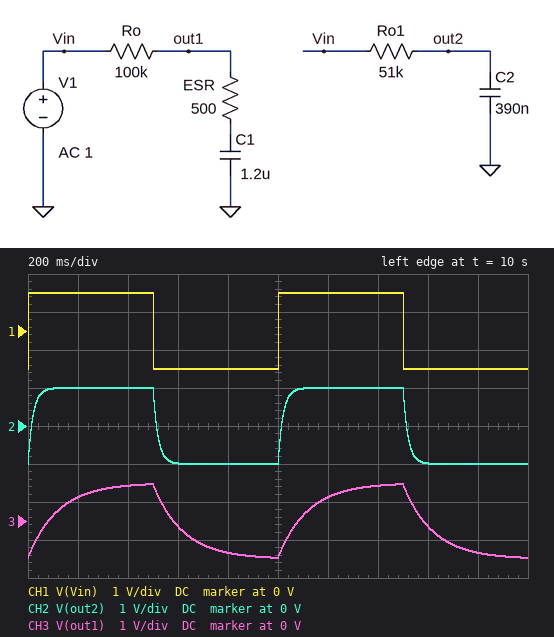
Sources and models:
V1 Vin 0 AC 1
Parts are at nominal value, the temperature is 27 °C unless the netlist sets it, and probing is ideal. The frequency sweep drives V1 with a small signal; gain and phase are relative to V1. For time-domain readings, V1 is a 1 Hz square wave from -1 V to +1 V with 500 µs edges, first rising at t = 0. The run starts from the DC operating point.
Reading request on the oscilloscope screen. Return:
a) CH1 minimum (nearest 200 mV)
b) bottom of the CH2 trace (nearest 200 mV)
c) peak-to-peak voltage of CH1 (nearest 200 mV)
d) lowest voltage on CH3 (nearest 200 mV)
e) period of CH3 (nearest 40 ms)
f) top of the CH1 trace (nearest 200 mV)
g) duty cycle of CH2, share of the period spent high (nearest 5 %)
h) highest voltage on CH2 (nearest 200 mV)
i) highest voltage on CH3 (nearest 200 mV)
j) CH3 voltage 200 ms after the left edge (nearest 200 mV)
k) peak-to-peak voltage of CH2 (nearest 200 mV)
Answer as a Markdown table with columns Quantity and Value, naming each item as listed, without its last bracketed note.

| Quantity | Value |
|---|---|
| CH1 minimum | -1.0 V |
| bottom of the CH2 trace | -1.0 V |
| peak-to-peak voltage of CH1 | 2.0 V |
| lowest voltage on CH3 | -1.0 V |
| period of CH3 | 1.00 s |
| top of the CH1 trace | 1.0 V |
| duty cycle of CH2, share of the period spent high | 50 % |
| highest voltage on CH2 | 1.0 V |
| highest voltage on CH3 | 1.0 V |
| CH3 voltage 200 ms after the left edge | 600 mV |
| peak-to-peak voltage of CH2 | 2.0 V |
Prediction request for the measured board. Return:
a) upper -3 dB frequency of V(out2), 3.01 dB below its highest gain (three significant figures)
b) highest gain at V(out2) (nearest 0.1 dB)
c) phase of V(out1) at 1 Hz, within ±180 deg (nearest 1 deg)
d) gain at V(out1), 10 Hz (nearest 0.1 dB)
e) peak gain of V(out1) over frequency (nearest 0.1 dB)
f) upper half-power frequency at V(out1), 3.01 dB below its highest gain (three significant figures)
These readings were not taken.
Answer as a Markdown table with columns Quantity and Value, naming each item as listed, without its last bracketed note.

| Quantity | Value |
|---|---|
| upper -3 dB frequency of V(out2), 3.01 dB below its highest gain | 8.00 Hz |
| highest gain at V(out2) | 0 dB |
| phase of V(out1) at 1 Hz, within ±180 deg | -37 deg |
| gain at V(out1), 10 Hz | -17.7 dB |
| peak gain of V(out1) over frequency | 0 dB |
| upper half-power frequency at V(out1), 3.01 dB below its highest gain | 1.32 Hz |
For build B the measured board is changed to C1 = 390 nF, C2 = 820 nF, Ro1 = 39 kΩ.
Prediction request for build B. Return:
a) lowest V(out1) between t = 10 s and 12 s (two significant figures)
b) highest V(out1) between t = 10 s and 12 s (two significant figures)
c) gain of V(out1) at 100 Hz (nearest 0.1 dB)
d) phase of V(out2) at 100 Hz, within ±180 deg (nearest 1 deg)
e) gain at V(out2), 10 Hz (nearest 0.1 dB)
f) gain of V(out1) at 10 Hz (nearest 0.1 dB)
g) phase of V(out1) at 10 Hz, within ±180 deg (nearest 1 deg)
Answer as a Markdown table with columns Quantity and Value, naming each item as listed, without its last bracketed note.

| Quantity | Value |
|---|---|
| lowest V(out1) between t = 10 s and 12 s | -1.0 V |
| highest V(out1) between t = 10 s and 12 s | 1.0 V |
| gain of V(out1) at 100 Hz | -27.8 dB |
| phase of V(out2) at 100 Hz, within ±180 deg | -87 deg |
| gain at V(out2), 10 Hz | -7.0 dB |
| gain of V(out1) at 10 Hz | -8.5 dB |
| phase of V(out1) at 10 Hz, within ±180 deg | -67 deg |
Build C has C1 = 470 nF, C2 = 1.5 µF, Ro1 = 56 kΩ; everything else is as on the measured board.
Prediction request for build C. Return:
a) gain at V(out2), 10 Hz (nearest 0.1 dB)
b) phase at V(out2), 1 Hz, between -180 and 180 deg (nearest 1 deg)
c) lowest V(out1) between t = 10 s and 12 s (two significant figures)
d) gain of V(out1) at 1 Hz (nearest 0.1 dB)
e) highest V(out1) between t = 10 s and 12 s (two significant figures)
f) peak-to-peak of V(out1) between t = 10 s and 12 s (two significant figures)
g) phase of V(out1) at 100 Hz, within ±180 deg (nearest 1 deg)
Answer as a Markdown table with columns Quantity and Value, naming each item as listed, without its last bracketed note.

| Quantity | Value |
|---|---|
| gain at V(out2), 10 Hz | -14.6 dB |
| phase at V(out2), 1 Hz, between -180 and 180 deg | -28 deg |
| lowest V(out1) between t = 10 s and 12 s | -1.0 V |
| gain of V(out1) at 1 Hz | -0.4 dB |
| highest V(out1) between t = 10 s and 12 s | 1.0 V |
| peak-to-peak of V(out1) between t = 10 s and 12 s | 2.0 V |
| phase of V(out1) at 100 Hz, within ±180 deg | -80 deg |
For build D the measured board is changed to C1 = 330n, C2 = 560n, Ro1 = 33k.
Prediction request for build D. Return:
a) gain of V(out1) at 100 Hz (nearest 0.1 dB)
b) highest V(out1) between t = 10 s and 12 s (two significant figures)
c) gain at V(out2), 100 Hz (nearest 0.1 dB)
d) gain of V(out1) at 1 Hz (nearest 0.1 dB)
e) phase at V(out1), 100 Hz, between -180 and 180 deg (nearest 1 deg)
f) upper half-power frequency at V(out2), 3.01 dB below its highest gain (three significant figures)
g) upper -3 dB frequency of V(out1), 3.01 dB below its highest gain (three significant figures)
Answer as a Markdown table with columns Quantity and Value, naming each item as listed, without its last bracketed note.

| Quantity | Value |
|---|---|
| gain of V(out1) at 100 Hz | -26.3 dB |
| highest V(out1) between t = 10 s and 12 s | 1.0 V |
| gain at V(out2), 100 Hz | -21.3 dB |
| gain of V(out1) at 1 Hz | -0.2 dB |
| phase at V(out1), 100 Hz, between -180 and 180 deg | -81 deg |
| upper half-power frequency at V(out2), 3.01 dB below its highest gain | 8.61 Hz |
| upper -3 dB frequency of V(out1), 3.01 dB below its highest gain | 4.80 Hz |
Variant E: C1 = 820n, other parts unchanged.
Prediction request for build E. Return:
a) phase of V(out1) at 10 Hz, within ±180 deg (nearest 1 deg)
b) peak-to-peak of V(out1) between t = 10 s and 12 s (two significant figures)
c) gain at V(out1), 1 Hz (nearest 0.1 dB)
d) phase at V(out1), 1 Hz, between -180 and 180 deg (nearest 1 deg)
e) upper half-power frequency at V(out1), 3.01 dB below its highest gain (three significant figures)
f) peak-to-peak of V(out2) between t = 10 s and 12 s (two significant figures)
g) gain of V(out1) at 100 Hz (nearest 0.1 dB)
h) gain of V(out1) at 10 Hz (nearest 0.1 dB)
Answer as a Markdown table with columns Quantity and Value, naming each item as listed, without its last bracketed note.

| Quantity | Value |
|---|---|
| phase of V(out1) at 10 Hz, within ±180 deg | -78 deg |
| peak-to-peak of V(out1) between t = 10 s and 12 s | 2.0 V |
| gain at V(out1), 1 Hz | -1.0 dB |
| phase at V(out1), 1 Hz, between -180 and 180 deg | -27 deg |
| upper half-power frequency at V(out1), 3.01 dB below its highest gain | 1.93 Hz |
| peak-to-peak of V(out2) between t = 10 s and 12 s | 2.0 V |
| gain of V(out1) at 100 Hz | -34.0 dB |
| gain of V(out1) at 10 Hz | -14.4 dB |
